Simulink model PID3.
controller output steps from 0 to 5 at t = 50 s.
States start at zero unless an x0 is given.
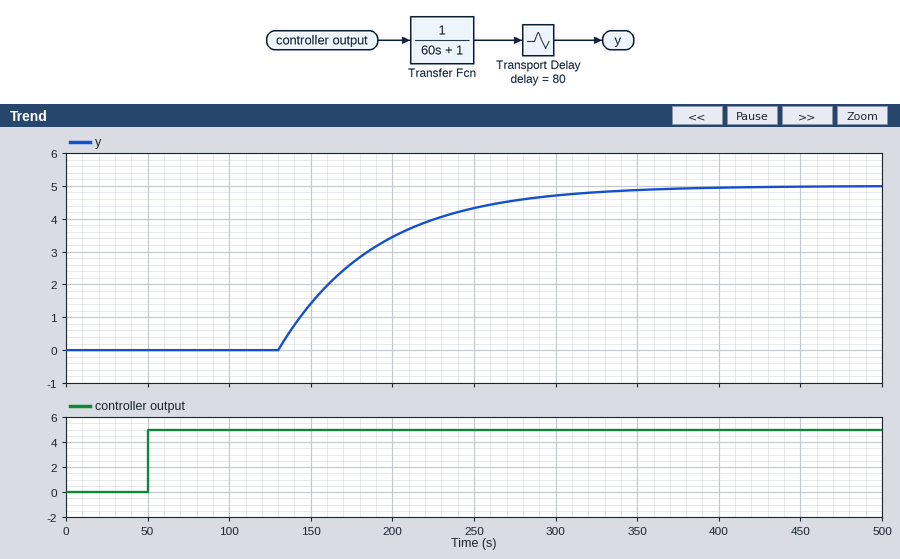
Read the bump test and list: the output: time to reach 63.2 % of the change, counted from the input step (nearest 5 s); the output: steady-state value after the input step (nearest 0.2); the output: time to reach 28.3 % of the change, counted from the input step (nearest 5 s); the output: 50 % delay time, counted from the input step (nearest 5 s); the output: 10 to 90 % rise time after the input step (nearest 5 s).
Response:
140 s
5.0
100 s
120 s
130 s
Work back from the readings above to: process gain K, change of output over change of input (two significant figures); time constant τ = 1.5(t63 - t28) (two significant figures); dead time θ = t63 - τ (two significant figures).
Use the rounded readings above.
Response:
1.0
60 s
80 s
